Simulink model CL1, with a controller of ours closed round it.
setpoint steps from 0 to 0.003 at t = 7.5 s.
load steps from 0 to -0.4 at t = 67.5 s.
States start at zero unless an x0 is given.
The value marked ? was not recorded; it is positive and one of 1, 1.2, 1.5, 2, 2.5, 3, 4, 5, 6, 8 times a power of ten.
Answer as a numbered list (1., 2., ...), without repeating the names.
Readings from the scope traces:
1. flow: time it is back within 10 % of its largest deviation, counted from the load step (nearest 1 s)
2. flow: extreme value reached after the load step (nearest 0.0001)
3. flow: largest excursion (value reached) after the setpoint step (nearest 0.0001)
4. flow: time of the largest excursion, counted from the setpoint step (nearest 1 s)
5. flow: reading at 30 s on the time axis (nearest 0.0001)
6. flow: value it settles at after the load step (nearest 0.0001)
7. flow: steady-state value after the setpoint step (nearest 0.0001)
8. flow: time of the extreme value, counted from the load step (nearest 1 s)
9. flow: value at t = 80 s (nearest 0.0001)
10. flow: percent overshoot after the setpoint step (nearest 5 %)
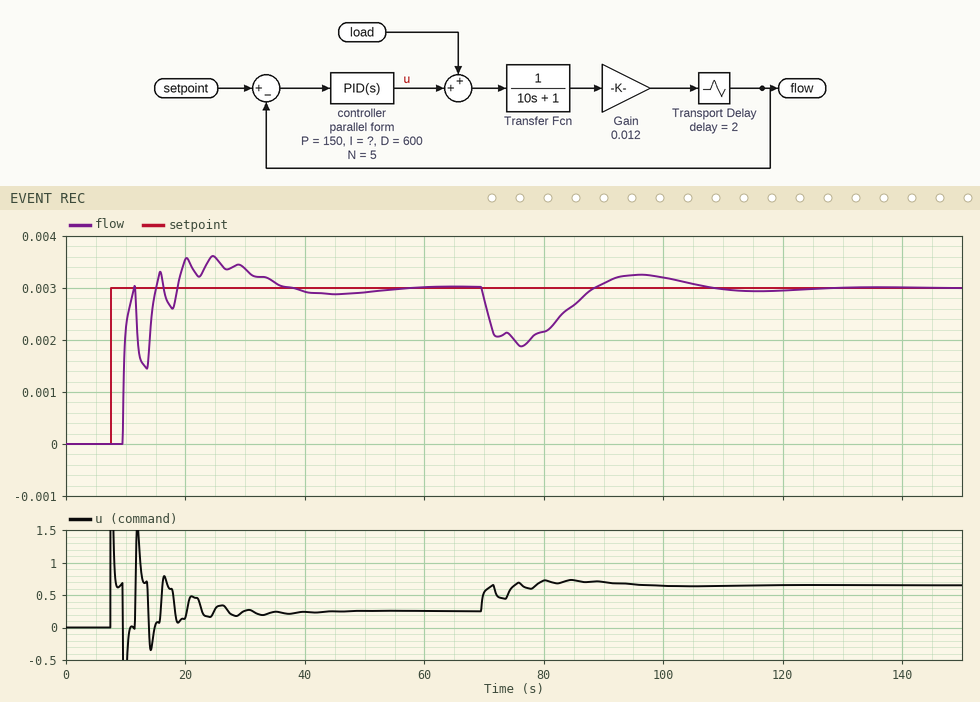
1. 36 s
2. 0.0019
3. 0.0036
4. 17 s
5. 0.0034
6. 0.0030
7. 0.0030
8. 9 s
9. 0.0022
10. 20 %
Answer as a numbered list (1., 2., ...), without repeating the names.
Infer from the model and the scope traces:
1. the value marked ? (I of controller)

1. 40
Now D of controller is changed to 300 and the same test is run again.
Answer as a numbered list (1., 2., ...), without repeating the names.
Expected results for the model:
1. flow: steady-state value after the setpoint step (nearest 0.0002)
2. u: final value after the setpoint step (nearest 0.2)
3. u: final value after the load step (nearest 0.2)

1. 0.0030
2. 0.2
3. 0.6
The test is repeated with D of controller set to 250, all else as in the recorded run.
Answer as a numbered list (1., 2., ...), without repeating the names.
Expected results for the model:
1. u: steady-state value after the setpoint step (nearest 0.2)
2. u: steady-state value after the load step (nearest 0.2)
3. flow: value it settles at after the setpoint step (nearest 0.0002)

1. 0.2
2. 0.6
3. 0.0030
